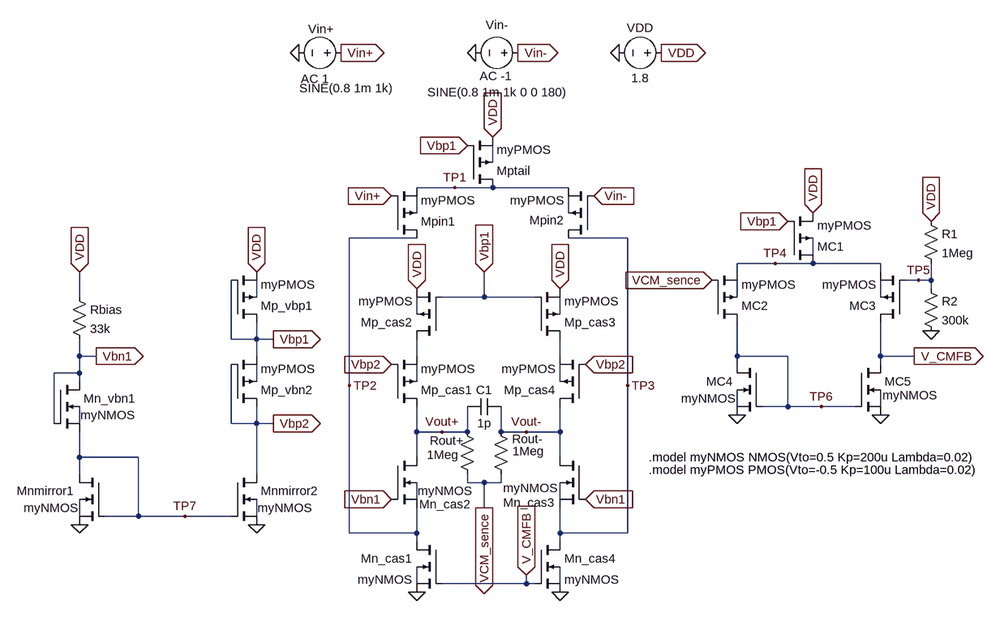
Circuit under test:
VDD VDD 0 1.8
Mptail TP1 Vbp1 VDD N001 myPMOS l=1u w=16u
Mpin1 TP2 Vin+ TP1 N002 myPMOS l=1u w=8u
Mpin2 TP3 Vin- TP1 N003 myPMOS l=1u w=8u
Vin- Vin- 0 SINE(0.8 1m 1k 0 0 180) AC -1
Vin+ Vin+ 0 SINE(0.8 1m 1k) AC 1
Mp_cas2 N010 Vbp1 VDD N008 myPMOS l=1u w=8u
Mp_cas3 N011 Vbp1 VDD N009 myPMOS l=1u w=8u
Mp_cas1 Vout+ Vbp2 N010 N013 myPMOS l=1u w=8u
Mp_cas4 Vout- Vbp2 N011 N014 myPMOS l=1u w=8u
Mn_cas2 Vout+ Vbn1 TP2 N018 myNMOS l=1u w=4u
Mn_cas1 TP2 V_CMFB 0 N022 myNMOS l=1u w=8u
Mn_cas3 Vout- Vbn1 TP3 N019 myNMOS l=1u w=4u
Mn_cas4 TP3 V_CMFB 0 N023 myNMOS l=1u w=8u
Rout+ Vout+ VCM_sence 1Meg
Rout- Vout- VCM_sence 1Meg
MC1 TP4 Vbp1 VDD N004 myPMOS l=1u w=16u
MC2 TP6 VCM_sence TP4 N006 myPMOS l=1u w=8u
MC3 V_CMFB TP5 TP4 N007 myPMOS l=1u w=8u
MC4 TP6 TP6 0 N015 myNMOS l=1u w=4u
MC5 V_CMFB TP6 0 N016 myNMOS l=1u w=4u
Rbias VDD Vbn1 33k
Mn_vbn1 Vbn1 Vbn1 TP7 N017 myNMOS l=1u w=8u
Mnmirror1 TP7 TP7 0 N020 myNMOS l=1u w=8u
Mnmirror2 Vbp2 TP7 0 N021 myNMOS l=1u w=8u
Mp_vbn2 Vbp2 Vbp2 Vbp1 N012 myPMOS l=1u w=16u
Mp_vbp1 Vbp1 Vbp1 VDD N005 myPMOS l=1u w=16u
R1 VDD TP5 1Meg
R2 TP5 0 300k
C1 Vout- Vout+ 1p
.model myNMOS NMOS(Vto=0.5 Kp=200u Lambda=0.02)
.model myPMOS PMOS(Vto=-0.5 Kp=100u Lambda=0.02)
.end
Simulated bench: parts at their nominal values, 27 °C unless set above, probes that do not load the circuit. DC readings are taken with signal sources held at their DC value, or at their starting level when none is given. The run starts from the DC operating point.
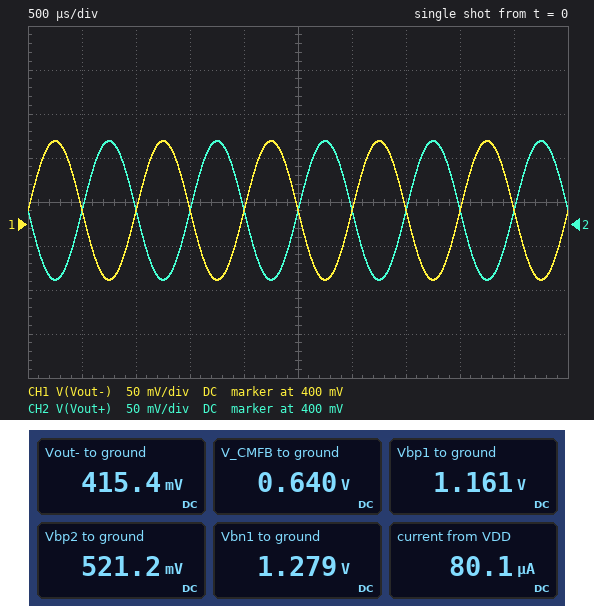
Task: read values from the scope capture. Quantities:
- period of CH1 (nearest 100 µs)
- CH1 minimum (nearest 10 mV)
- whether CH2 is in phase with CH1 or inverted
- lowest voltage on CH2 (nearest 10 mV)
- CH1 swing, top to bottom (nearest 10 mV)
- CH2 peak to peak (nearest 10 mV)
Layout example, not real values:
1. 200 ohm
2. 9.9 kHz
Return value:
1. 1.0 ms
2. 340 mV
3. inverted
4. 340 mV
5. 160 mV
6. 160 mV
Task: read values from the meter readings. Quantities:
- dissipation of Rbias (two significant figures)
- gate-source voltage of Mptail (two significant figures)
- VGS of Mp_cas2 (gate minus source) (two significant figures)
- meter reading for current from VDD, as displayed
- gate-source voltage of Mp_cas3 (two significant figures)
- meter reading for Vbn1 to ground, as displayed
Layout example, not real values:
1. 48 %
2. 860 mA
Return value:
1. 8.2 µW
2. -640 mV
3. -640 mV
4. 80.1 µA
5. -640 mV
6. 1.279 V
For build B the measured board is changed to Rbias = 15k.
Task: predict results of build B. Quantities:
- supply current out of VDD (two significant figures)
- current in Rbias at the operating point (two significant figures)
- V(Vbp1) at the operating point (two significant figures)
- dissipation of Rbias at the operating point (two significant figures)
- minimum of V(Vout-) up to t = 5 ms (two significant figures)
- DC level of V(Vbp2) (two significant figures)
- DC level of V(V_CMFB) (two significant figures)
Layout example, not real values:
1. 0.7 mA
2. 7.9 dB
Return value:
1. 140 µA
2. 28 µA
3. 1.1 V
4. 12 µW
5. 330 mV
6. 430 mV
7. 690 mV
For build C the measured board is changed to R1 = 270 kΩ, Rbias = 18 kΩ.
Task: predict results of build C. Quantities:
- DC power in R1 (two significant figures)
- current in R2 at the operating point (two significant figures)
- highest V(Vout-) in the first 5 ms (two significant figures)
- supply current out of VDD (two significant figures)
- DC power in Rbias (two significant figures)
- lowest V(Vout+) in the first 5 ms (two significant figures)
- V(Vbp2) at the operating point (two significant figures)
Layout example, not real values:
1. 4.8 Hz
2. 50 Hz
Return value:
1. 2.7 µW
2. 3.2 µA
3. 1.1 V
4. 130 µA
5. 11 µW
6. 810 mV
7. 450 mV
